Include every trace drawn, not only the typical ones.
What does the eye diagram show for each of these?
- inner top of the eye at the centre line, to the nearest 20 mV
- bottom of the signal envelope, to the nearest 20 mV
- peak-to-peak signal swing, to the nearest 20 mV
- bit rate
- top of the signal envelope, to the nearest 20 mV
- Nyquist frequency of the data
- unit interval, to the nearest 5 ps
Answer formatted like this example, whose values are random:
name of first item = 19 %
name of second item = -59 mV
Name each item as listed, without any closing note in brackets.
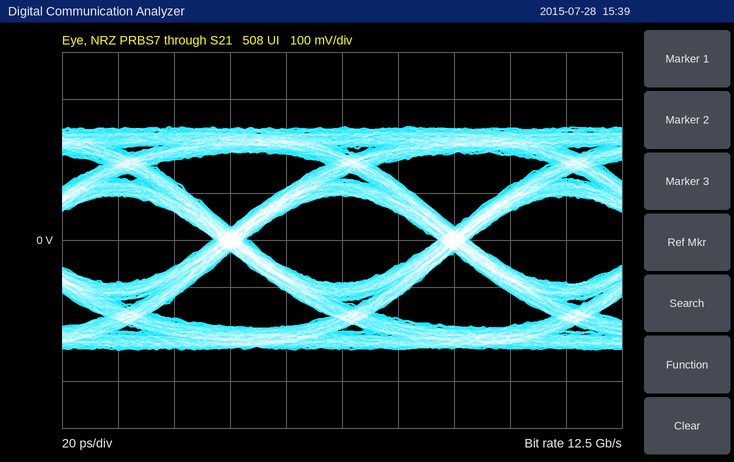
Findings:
inner top of the eye at the centre line, to the nearest 20 mV = 100 mV
bottom of the signal envelope, to the nearest 20 mV = -240 mV
peak-to-peak signal swing, to the nearest 20 mV = 480 mV
bit rate = 12.5 Gb/s
top of the signal envelope, to the nearest 20 mV = 240 mV
Nyquist frequency of the data = 6.25 GHz
unit interval, to the nearest 5 ps = 80 ps
